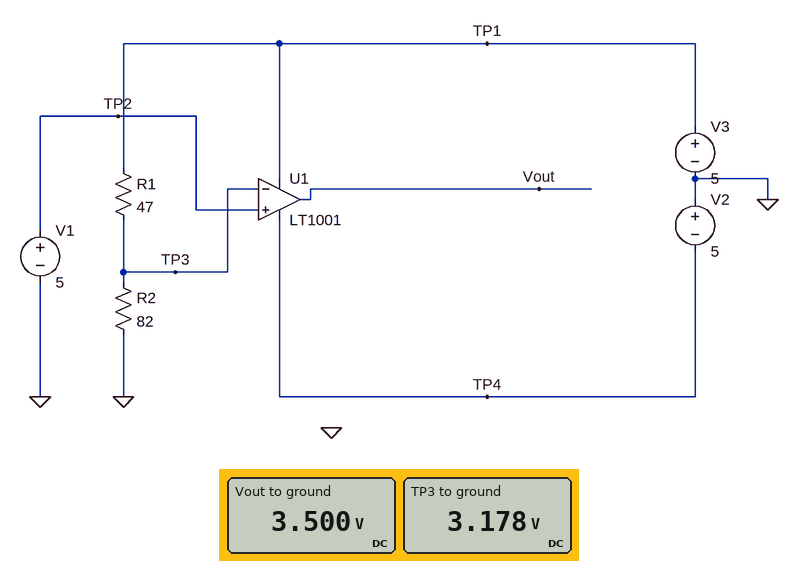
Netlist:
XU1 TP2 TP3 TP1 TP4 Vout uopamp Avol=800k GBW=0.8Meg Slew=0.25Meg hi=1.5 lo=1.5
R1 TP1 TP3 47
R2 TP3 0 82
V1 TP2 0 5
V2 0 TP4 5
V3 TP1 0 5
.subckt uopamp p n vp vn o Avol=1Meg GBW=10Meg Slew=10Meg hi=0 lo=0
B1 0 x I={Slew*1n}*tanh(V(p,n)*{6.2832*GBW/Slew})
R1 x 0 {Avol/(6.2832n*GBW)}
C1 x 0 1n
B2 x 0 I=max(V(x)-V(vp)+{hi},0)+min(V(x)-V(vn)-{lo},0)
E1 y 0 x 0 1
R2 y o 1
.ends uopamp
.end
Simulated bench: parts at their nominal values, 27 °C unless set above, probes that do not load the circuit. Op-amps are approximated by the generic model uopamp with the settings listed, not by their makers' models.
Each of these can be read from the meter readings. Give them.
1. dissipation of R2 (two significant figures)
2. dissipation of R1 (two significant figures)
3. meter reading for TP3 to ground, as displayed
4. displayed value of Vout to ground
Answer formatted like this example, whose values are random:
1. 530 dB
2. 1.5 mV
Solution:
1. 120 mW
2. 71 mW
3. 3.178 V
4. 3.500 V
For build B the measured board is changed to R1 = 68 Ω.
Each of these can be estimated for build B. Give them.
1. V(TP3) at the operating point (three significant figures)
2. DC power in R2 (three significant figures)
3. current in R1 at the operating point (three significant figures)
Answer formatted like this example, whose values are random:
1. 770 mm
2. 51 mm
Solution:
1. 2.73 V
2. 91.1 mW
3. 33.3 mA
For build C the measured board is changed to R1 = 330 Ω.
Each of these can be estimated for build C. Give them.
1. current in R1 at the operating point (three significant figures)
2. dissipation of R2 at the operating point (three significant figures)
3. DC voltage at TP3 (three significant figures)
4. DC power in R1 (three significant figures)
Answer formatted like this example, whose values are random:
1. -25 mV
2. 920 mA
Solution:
1. 12.1 mA
2. 12.1 mW
3. 995 mV
4. 48.6 mW
